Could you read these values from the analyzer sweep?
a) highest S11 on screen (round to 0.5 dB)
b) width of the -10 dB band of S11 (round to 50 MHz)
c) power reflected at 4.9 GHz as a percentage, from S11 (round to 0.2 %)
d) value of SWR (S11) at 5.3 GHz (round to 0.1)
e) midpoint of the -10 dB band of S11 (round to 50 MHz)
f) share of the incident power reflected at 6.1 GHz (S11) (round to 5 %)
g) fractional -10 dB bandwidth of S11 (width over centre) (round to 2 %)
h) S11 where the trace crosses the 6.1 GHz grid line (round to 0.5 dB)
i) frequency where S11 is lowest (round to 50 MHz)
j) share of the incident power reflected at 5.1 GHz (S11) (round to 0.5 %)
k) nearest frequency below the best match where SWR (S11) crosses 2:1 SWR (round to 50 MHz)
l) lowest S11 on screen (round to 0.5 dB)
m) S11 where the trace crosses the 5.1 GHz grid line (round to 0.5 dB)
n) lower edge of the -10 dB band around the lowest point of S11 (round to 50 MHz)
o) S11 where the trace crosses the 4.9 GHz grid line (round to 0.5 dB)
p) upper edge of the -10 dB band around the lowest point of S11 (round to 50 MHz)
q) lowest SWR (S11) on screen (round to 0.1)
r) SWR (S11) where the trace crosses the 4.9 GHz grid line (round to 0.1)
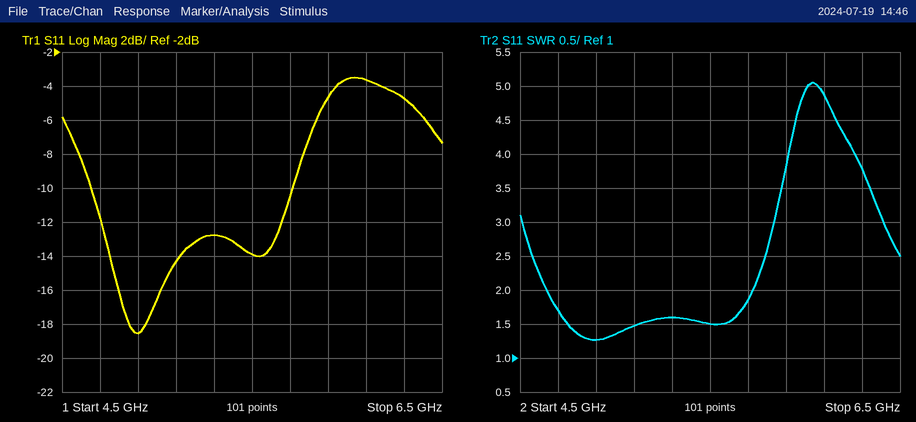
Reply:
-3.5 dB
1.05 GHz
1.4 %
1.6
5.20 GHz
45 %
20 %
-3.5 dB
4.90 GHz
3.5 %
4.65 GHz
-18.5 dB
-14.5 dB
4.65 GHz
-18.5 dB
5.70 GHz
1.3
1.3
